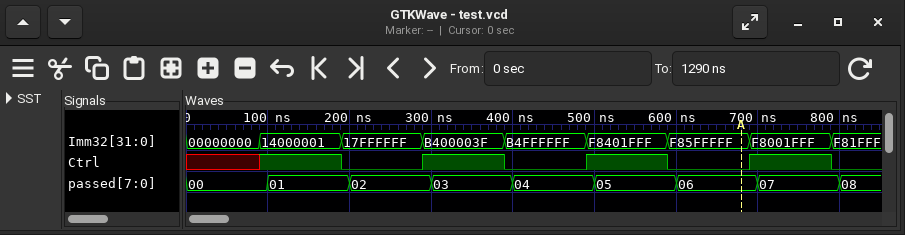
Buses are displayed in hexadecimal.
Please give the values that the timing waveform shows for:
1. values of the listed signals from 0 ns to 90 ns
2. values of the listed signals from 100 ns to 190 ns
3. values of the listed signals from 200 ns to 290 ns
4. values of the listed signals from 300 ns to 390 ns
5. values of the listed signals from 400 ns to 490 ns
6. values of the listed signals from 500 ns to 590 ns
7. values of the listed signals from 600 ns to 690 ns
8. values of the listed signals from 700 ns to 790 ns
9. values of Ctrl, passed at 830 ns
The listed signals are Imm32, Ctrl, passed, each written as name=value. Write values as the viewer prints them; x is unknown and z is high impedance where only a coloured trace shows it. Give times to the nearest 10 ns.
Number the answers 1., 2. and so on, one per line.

1. Imm32=00000000, Ctrl=x, passed=00
2. Imm32=14000001, Ctrl=1, passed=01
3. Imm32=17FFFFFF, Ctrl=0, passed=02
4. Imm32=B400003F, Ctrl=1, passed=03
5. Imm32=B4FFFFFF, Ctrl=0, passed=04
6. Imm32=F8401FFF, Ctrl=1, passed=05
7. Imm32=F85FFFFF, Ctrl=0, passed=06
8. Imm32=F8001FFF, Ctrl=1, passed=07
9. Ctrl=0, passed=08
